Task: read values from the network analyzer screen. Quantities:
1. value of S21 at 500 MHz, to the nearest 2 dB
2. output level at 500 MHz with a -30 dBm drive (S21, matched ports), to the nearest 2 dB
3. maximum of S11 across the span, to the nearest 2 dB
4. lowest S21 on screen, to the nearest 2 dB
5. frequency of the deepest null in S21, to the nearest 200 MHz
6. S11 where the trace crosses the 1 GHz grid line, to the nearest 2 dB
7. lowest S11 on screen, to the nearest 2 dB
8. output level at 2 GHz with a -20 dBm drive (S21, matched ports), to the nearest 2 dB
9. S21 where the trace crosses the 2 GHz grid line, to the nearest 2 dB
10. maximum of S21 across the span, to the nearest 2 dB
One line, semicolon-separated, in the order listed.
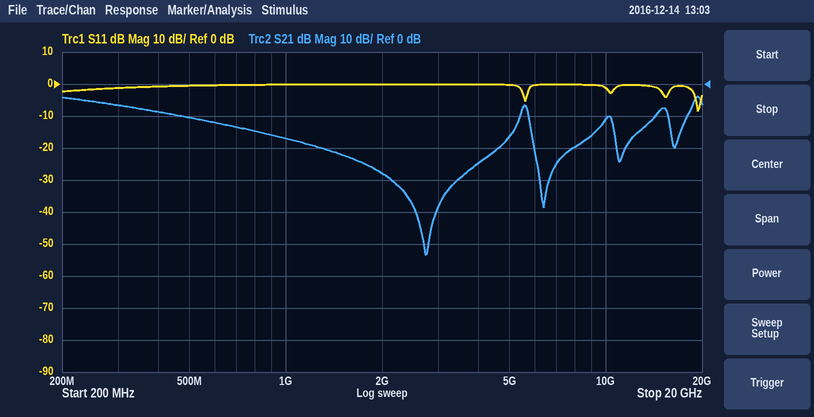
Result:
-10 dB; -40 dBm; 0 dB; -54 dB; 2.8 GHz; 0 dB; -8 dB; -48 dBm; -28 dB; -4 dB
